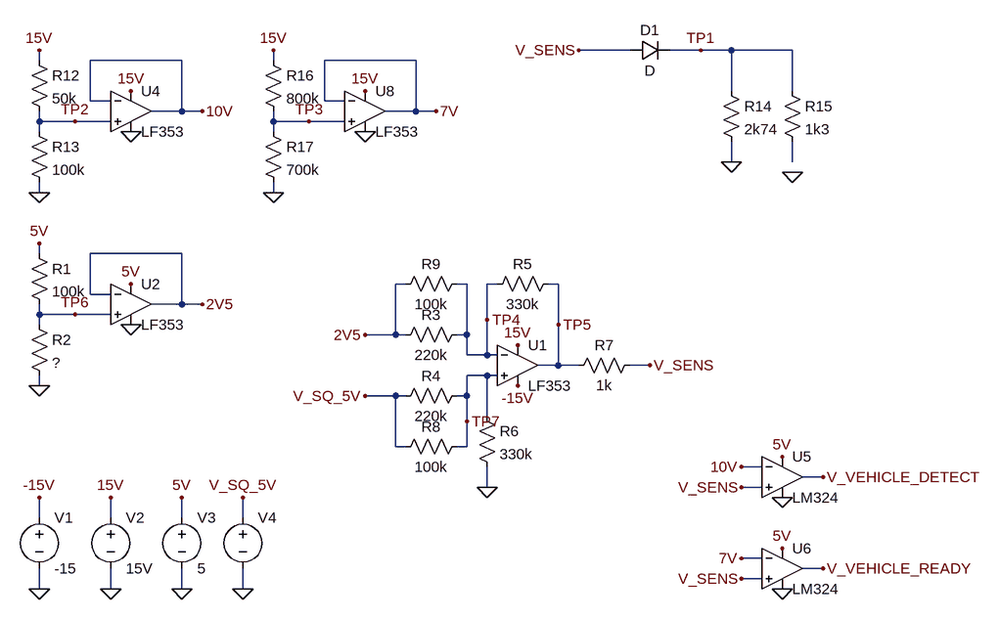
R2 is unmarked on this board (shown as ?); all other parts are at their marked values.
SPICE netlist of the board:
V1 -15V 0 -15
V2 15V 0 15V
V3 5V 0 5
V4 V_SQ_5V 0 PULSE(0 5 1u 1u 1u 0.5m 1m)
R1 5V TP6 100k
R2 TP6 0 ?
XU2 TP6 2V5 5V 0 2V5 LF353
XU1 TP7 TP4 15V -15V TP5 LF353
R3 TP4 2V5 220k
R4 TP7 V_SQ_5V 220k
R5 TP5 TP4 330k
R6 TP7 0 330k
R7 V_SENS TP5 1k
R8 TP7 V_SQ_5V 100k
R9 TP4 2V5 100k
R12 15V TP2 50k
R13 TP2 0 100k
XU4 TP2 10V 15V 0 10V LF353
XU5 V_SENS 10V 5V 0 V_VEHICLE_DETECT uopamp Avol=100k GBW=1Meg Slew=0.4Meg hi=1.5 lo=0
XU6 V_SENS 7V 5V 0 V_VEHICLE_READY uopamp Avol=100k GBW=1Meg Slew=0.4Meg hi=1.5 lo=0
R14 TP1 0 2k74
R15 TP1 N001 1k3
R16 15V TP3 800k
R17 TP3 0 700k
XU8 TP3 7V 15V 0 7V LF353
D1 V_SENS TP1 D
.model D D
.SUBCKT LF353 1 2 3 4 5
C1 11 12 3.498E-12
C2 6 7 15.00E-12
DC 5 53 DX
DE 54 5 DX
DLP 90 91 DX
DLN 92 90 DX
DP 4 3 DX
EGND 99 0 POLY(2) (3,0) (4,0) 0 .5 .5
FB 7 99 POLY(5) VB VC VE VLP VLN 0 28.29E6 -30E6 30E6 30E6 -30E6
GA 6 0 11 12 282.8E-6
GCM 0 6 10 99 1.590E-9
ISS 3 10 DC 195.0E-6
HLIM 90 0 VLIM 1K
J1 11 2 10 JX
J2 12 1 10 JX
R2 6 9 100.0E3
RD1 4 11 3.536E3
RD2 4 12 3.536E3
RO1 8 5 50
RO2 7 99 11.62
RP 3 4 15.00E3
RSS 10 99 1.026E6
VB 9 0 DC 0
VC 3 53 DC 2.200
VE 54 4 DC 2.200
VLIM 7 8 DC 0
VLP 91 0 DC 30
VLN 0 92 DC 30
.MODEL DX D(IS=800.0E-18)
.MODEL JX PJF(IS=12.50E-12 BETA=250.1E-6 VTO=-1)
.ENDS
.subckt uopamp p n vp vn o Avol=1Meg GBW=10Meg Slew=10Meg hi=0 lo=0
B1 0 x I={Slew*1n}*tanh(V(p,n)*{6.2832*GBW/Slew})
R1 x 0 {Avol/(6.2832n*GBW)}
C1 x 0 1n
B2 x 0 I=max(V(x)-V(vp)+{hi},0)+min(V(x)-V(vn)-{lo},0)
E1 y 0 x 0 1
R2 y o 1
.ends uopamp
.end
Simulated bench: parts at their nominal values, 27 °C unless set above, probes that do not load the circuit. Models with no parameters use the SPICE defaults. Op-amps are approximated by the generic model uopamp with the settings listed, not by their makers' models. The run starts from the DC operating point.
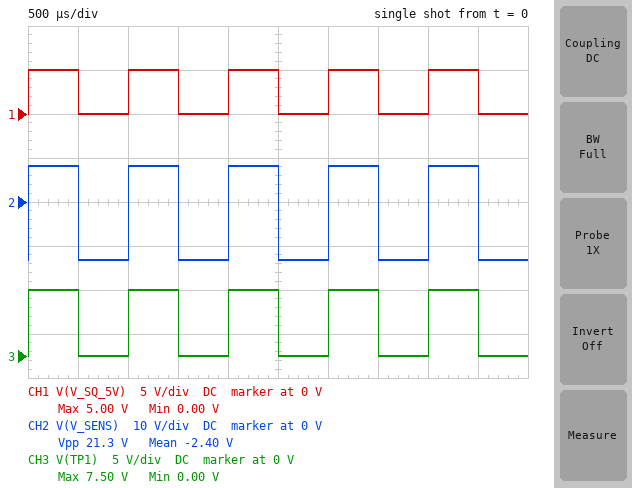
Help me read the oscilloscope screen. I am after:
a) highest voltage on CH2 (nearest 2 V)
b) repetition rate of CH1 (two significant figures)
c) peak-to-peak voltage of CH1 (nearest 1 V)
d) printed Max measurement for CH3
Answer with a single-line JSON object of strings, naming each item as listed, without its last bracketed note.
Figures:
{"highest voltage on CH2": "8 V", "repetition rate of CH1": "1.0 kHz", "peak-to-peak voltage of CH1": "5 V", "printed Max measurement for CH3": "7.50 V"}
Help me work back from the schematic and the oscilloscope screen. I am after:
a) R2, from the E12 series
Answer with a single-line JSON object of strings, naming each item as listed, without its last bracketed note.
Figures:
{"R2, from the E12 series": "120 kΩ"}
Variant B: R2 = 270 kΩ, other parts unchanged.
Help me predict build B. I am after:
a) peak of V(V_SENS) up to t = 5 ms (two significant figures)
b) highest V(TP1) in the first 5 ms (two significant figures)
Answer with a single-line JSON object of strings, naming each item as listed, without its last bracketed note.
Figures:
{"peak of V(V_SENS) up to t = 5 ms": "5.6 V", "highest V(TP1) in the first 5 ms": "5.0 V"}
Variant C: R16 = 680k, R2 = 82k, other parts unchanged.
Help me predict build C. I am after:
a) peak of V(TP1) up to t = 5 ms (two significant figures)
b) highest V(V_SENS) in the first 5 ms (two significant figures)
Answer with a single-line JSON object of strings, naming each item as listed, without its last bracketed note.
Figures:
{"peak of V(TP1) up to t = 5 ms": "9.2 V", "highest V(V_SENS) in the first 5 ms": "9.8 V"}
